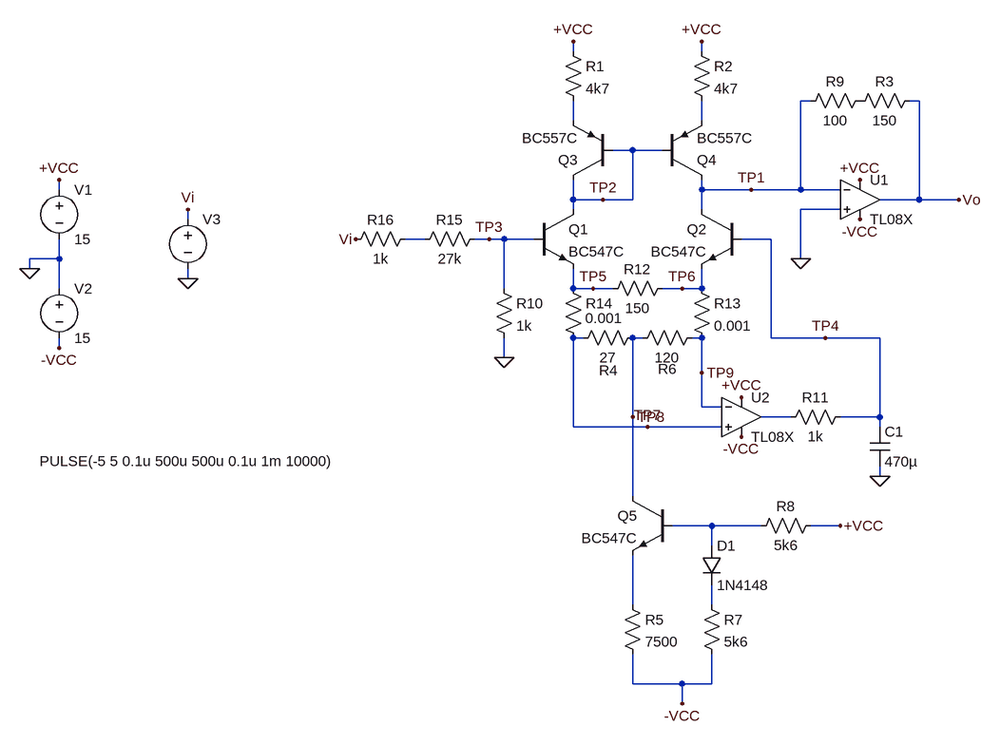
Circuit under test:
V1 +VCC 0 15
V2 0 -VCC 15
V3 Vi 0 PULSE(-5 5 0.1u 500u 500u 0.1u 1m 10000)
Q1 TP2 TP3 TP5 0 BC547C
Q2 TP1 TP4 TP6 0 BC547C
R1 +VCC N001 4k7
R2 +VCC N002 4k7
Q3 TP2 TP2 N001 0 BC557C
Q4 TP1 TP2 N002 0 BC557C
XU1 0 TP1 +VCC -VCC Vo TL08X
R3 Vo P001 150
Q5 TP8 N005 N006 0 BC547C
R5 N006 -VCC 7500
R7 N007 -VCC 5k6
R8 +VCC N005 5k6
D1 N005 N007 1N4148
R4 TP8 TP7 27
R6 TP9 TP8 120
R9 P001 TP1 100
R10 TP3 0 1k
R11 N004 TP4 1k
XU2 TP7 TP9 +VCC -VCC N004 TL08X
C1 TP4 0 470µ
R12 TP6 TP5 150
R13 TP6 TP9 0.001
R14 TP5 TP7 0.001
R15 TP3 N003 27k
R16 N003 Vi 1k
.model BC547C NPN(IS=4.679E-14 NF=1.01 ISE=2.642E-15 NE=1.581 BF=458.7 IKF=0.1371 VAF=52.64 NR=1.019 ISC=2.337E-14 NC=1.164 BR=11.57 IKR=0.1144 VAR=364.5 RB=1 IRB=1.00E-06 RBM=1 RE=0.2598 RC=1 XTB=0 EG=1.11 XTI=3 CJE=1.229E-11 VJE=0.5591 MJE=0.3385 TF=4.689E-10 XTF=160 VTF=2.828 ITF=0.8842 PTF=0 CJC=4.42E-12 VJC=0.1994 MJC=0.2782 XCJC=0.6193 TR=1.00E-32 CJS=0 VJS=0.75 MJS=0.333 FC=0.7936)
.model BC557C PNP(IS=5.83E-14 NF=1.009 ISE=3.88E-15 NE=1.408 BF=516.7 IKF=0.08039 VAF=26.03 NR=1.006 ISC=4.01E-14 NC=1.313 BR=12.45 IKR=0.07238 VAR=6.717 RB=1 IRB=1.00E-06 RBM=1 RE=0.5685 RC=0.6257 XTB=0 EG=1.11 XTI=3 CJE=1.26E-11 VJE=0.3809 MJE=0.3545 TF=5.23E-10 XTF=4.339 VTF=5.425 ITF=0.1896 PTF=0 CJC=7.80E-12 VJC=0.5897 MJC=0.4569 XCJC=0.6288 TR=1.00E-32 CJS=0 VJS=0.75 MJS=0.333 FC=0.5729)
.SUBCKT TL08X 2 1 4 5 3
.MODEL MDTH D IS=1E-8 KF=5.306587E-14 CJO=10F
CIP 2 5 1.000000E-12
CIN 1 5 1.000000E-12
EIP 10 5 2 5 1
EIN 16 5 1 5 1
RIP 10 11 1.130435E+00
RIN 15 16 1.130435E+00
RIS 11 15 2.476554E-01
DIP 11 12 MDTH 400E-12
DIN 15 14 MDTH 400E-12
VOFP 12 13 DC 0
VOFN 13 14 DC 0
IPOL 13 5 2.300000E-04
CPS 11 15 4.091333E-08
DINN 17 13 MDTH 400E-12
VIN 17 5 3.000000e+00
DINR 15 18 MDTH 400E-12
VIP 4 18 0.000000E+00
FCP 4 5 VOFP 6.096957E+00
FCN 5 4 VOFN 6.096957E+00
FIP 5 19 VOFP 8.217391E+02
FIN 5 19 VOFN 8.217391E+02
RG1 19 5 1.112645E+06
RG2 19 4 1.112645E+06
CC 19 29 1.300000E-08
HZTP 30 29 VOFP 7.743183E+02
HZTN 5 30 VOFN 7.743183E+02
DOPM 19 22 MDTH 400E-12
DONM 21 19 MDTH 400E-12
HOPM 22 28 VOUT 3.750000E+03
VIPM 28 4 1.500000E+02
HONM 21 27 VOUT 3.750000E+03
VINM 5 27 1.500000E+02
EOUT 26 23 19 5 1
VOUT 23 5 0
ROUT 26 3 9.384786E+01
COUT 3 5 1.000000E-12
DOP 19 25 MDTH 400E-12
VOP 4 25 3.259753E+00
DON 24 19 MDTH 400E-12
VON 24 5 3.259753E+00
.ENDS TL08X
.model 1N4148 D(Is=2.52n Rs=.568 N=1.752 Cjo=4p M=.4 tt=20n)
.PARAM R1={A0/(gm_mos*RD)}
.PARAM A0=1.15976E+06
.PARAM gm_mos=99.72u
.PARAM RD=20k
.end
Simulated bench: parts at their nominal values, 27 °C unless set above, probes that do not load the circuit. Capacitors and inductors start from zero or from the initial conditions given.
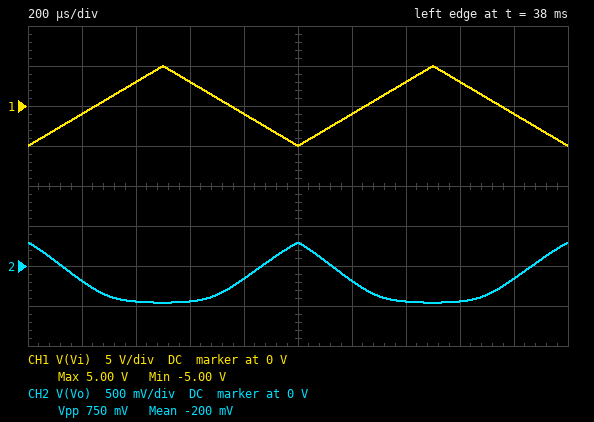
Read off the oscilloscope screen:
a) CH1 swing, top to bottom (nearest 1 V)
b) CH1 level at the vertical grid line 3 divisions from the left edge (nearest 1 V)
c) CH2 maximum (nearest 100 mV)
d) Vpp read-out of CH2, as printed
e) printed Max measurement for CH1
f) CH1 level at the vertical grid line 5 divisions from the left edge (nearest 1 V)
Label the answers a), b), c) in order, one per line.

a) 10 V
b) 3 V
c) 300 mV
d) 750 mV
e) 5.00 V
f) -5 V
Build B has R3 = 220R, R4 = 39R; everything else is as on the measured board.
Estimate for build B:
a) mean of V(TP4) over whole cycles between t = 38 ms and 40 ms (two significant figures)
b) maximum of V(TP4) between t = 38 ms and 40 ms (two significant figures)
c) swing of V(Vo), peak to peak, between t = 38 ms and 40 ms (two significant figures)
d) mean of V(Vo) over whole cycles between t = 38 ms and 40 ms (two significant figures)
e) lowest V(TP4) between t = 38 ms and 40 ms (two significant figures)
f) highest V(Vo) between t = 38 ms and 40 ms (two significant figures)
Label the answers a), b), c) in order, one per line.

a) -29 mV
b) -23 mV
c) 1.0 V
d) -210 mV
e) -35 mV
f) 420 mV
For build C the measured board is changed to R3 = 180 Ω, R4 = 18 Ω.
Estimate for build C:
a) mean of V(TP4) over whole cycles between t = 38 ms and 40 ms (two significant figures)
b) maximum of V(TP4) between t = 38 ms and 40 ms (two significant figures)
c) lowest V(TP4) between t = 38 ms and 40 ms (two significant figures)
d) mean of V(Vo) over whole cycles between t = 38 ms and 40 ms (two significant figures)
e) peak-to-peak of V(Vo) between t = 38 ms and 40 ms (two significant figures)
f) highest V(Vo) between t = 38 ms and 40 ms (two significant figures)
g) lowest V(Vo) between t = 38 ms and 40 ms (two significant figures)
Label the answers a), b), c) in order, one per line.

a) -53 mV
b) -47 mV
c) -58 mV
d) -270 mV
e) 790 mV
f) 280 mV
g) -520 mV
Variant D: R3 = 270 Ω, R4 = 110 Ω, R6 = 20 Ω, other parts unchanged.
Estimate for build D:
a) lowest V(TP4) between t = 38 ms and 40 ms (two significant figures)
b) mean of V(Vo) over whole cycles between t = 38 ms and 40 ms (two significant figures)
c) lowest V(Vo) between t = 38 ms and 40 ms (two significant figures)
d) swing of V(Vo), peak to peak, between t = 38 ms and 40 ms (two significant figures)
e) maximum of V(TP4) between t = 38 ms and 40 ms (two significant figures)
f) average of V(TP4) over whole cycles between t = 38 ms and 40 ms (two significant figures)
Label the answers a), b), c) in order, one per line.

a) 47 mV
b) 330 mV
c) -420 mV
d) 1.1 V
e) 58 mV
f) 53 mV
